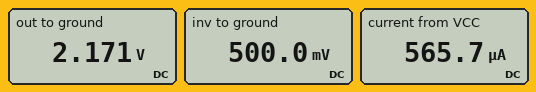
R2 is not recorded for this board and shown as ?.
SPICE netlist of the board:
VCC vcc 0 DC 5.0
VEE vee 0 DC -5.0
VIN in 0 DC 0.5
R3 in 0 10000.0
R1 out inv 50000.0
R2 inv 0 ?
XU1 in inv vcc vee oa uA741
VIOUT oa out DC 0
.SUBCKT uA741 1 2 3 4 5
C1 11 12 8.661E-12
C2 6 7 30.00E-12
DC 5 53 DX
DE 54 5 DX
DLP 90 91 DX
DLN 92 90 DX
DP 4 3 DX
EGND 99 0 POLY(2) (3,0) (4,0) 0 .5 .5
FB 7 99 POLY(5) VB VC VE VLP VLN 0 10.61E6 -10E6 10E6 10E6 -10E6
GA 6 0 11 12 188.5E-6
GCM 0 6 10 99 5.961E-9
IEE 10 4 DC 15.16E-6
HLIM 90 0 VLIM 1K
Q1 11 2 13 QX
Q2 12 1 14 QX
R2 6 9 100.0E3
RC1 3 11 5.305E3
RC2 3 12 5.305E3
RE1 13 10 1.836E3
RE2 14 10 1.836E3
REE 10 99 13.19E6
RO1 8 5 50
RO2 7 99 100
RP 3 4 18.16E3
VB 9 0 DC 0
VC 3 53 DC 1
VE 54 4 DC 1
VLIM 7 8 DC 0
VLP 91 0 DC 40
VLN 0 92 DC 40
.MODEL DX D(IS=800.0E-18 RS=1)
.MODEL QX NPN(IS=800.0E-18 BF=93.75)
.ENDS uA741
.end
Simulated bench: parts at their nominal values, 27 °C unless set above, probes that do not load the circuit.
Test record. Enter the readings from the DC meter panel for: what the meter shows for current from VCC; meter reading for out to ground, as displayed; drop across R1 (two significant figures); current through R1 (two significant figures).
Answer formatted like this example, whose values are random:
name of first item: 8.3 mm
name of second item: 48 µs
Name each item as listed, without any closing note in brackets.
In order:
what the meter shows for current from VCC: 565.7 µA
meter reading for out to ground, as displayed: 2.171 V
drop across R1: 1.7 V
current through R1: 33 µA
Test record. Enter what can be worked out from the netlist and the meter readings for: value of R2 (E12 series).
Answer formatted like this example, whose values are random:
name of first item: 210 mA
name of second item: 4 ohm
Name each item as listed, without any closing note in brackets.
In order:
value of R2: 15 kΩ
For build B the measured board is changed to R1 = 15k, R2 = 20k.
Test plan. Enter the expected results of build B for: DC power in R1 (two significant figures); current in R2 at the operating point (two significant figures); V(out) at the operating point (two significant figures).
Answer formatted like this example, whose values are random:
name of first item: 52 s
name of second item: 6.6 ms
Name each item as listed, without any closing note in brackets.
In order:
DC power in R1: 9.4 µW
current in R2 at the operating point: 25 µA
V(out) at the operating point: 880 mV
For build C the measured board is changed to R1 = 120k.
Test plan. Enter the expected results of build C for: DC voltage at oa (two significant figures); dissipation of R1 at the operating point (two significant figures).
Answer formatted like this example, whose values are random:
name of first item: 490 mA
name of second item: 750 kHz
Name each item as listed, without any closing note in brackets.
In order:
DC voltage at oa: 4.5 V
dissipation of R1 at the operating point: 130 µW
